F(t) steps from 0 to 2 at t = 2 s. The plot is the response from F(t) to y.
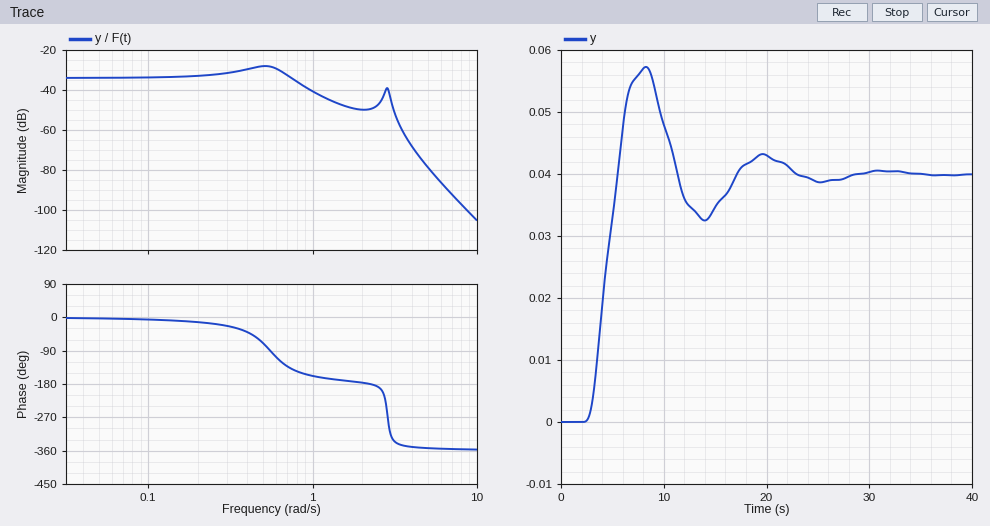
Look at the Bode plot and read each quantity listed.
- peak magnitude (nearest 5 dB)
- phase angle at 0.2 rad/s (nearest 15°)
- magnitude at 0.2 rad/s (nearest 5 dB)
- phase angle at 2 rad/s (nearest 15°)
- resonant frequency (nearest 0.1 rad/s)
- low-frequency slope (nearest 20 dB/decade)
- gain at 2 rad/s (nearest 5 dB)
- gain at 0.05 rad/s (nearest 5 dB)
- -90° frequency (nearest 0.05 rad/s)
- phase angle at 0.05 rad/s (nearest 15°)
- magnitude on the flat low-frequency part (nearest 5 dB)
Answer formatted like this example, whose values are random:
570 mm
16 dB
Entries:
-30 dB
-15°
-35 dB
-180°
0.5 rad/s
0 dB/decade
-50 dB
-35 dB
0.55 rad/s
0°
-35 dB
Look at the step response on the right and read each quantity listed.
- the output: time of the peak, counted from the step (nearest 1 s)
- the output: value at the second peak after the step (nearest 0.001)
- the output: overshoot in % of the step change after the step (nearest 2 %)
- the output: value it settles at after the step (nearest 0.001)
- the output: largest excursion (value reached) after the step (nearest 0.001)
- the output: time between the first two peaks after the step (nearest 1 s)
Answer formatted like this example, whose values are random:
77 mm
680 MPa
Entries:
6 s
0.043
44 %
0.040
0.057
11 s
